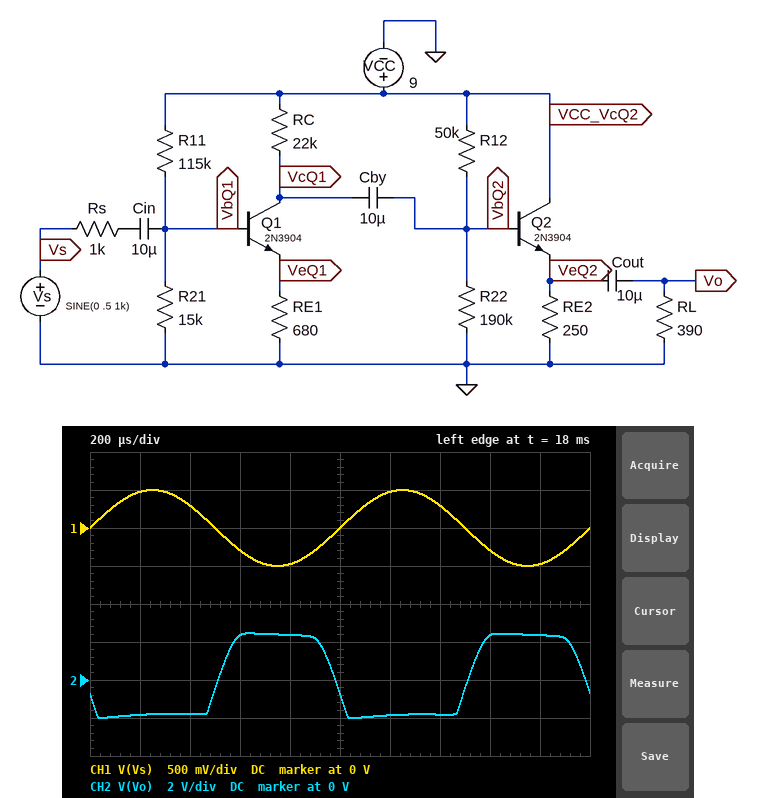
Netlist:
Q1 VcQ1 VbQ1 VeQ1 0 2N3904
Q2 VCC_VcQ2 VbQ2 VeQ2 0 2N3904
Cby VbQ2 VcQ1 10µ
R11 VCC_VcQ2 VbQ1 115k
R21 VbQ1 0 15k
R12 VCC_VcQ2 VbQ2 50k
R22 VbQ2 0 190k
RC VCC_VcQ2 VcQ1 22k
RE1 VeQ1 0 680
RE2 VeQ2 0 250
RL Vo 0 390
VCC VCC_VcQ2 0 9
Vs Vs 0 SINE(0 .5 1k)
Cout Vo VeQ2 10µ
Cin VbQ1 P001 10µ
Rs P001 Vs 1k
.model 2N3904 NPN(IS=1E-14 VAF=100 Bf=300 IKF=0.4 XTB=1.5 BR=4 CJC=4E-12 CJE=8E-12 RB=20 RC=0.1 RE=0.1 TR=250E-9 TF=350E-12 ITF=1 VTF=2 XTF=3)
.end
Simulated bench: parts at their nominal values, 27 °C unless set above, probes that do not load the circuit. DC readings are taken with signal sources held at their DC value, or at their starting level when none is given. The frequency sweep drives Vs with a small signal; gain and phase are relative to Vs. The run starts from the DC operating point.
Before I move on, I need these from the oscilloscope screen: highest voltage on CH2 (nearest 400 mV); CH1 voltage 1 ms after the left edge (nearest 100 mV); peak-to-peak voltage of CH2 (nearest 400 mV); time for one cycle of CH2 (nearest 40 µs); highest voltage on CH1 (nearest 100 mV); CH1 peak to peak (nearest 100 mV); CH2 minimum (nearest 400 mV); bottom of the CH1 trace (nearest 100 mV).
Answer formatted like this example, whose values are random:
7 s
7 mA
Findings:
2.4 V
0 V
4.4 V
1.00 ms
500 mV
1.0 V
-2.0 V
-500 mV
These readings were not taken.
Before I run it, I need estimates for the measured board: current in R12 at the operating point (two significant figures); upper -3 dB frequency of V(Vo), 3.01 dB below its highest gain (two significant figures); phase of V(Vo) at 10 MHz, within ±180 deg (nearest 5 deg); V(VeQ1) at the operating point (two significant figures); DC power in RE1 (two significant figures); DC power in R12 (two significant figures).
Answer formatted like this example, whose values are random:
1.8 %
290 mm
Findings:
82 µA
250 kHz
-5 deg
270 mV
110 µW
330 µW
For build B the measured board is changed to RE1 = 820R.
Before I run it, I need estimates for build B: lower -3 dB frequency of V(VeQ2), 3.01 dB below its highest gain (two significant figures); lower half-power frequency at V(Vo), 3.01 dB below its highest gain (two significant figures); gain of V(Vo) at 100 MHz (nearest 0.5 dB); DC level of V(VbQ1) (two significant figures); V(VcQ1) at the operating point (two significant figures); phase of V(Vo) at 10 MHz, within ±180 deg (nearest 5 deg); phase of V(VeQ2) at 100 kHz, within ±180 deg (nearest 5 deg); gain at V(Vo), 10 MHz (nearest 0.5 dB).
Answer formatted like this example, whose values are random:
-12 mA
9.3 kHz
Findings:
6.7 Hz
41 Hz
-12.5 dB
960 mV
410 mV
0 deg
145 deg
-7.5 dB
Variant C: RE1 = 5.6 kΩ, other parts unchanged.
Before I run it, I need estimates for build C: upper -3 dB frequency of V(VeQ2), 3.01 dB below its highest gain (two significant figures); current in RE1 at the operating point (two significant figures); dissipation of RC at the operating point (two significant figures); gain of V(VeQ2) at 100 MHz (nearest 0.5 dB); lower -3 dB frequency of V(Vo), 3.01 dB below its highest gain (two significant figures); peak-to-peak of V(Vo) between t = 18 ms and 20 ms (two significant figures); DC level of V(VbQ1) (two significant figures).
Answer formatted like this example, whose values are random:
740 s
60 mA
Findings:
1.8 MHz
80 µA
140 µW
-14.0 dB
37 Hz
1.6 V
1.0 V
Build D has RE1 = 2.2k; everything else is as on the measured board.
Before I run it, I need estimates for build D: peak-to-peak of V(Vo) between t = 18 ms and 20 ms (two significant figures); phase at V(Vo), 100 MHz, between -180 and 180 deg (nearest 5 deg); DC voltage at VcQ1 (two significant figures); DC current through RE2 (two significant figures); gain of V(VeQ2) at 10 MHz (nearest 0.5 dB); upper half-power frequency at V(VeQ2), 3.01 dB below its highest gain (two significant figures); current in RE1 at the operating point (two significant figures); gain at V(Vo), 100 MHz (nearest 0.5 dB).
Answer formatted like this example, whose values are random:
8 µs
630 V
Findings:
4.0 V
-25 deg
4.8 V
17 mA
-1.5 dB
1.6 MHz
190 µA
-14.0 dB
